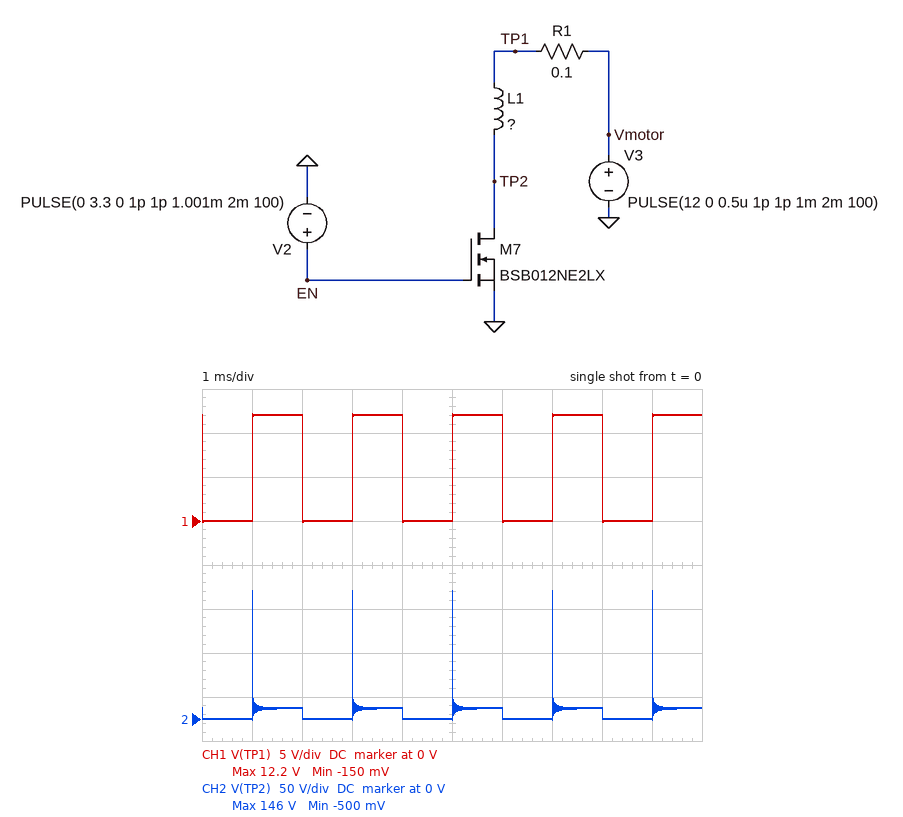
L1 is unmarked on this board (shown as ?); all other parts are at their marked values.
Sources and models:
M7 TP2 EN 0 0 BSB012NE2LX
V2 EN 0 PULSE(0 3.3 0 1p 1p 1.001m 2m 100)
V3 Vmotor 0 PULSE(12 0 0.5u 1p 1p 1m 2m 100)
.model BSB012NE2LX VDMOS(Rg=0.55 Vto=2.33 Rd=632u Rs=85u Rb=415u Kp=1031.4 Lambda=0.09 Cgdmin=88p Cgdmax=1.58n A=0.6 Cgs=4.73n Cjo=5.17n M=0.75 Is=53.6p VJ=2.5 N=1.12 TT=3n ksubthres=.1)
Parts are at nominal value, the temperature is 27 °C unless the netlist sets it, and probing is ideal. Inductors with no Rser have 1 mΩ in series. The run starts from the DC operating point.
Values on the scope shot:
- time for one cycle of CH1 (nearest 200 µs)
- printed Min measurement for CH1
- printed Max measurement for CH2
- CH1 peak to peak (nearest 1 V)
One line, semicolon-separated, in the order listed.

2.0 ms; -150 mV; 146 V; 12 V
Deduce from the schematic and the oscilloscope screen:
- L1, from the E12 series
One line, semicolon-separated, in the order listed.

4.7 µH
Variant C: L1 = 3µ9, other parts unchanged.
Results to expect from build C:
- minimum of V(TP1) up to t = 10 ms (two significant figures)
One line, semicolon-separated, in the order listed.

-150 mV
